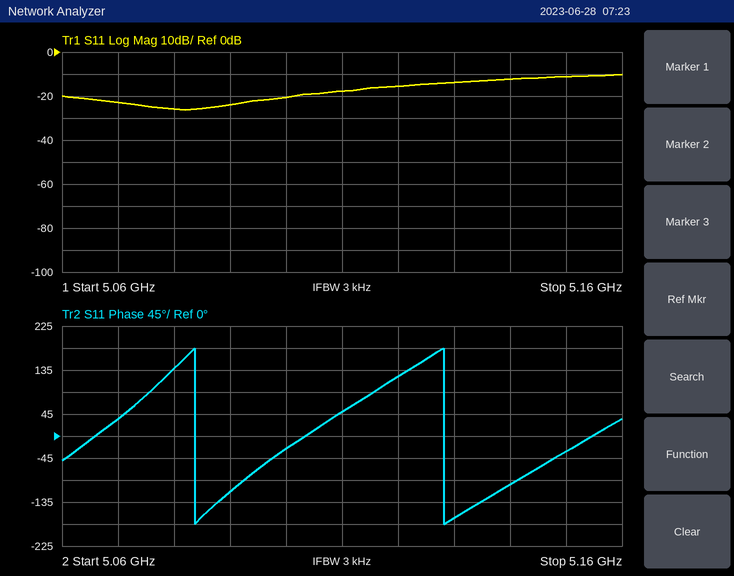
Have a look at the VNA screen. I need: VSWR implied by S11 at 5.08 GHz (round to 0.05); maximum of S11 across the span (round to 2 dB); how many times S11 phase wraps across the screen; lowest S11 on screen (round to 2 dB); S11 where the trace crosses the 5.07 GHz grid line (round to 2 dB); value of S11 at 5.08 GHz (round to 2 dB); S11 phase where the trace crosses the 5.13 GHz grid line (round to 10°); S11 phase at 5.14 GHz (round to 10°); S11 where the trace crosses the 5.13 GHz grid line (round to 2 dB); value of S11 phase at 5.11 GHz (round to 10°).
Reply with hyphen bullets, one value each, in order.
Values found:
- 1.10
- -10 dB
- 2
- -26 dB
- -22 dB
- -26 dB
- -170°
- -100°
- -14 dB
- 50°
